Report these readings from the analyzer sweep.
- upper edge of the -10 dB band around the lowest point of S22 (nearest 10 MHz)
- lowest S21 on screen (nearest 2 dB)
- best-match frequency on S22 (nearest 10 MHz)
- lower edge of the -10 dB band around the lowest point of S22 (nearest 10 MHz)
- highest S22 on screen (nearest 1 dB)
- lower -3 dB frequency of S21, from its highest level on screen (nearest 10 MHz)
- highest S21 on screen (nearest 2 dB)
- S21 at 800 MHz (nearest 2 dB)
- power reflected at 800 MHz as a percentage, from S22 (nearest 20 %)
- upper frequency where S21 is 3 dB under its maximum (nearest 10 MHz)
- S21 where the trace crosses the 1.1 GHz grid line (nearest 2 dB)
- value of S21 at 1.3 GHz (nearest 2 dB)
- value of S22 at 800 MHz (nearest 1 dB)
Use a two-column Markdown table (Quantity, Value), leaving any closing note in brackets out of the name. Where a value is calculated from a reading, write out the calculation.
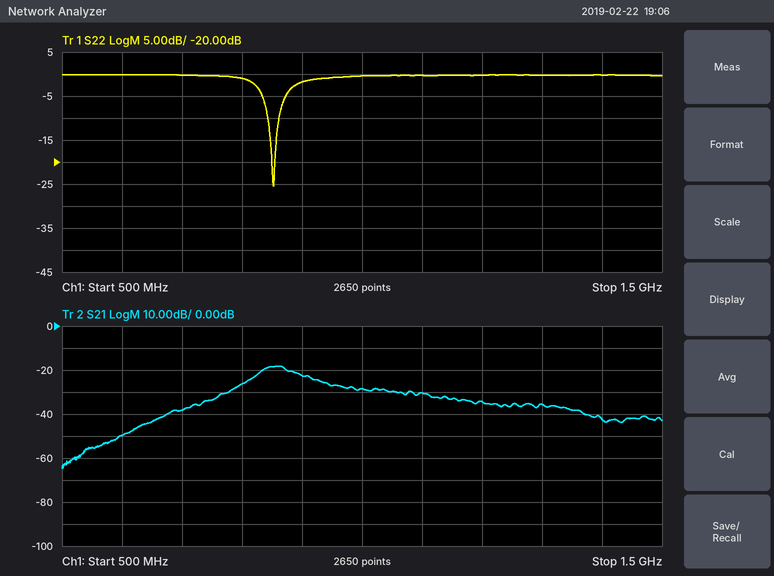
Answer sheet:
| Quantity | Value |
|---|---|
| upper edge of the -10 dB band around the lowest point of S22 | 860 MHz |
| lowest S21 on screen | -64 dB |
| best-match frequency on S22 | 850 MHz |
| lower edge of the -10 dB band around the lowest point of S22 | 840 MHz |
| highest S22 on screen | 0 dB |
| lower -3 dB frequency of S21, from its highest level on screen | 830 MHz |
| highest S21 on screen | -18 dB |
| S21 at 800 MHz | -26 dB |
| power reflected at 800 MHz as a percentage, from S22 | 10^(-1/10) ≈ 79.4 %, so 80 % to the nearest 20 % |
| upper frequency where S21 is 3 dB under its maximum | 890 MHz |
| S21 where the trace crosses the 1.1 GHz grid line | -30 dB |
| value of S21 at 1.3 GHz | -36 dB |
| value of S22 at 800 MHz | -1 dB |
